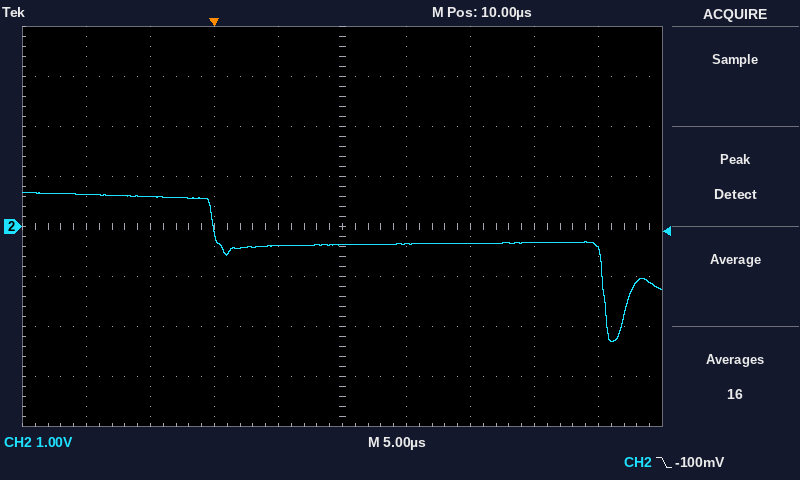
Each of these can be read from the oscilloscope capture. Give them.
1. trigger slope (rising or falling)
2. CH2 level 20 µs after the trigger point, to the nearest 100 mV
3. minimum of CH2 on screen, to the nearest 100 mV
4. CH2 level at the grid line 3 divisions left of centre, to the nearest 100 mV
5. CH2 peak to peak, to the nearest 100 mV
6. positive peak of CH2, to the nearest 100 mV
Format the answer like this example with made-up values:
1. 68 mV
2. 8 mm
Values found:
1. falling
2. -300 mV
3. -2.3 V
4. 600 mV
5. 3.0 V
6. 700 mV
